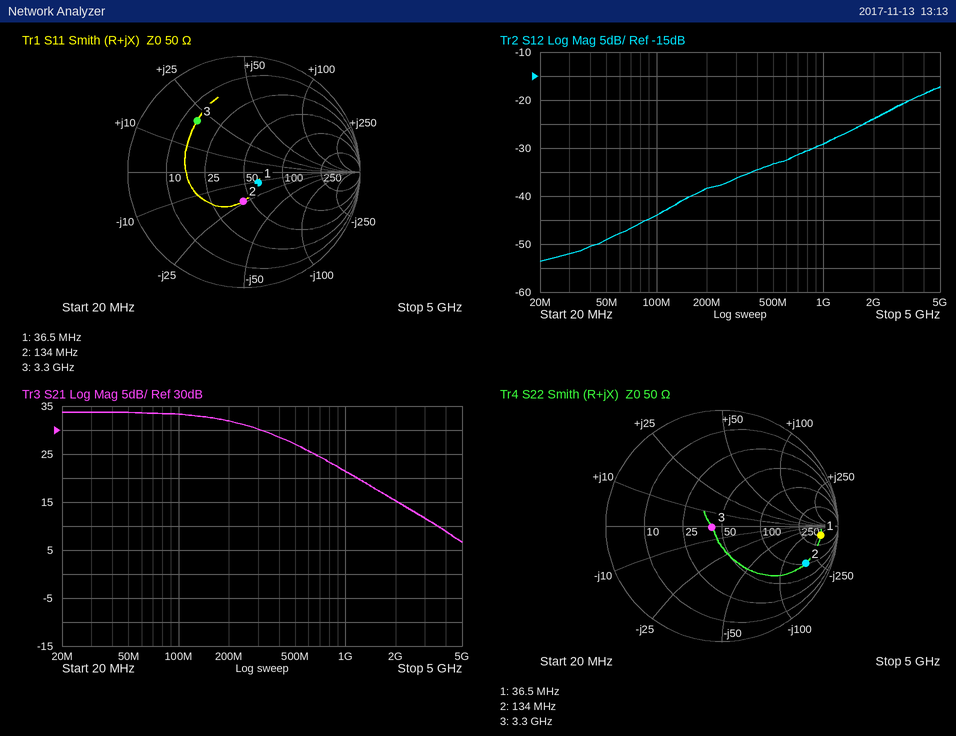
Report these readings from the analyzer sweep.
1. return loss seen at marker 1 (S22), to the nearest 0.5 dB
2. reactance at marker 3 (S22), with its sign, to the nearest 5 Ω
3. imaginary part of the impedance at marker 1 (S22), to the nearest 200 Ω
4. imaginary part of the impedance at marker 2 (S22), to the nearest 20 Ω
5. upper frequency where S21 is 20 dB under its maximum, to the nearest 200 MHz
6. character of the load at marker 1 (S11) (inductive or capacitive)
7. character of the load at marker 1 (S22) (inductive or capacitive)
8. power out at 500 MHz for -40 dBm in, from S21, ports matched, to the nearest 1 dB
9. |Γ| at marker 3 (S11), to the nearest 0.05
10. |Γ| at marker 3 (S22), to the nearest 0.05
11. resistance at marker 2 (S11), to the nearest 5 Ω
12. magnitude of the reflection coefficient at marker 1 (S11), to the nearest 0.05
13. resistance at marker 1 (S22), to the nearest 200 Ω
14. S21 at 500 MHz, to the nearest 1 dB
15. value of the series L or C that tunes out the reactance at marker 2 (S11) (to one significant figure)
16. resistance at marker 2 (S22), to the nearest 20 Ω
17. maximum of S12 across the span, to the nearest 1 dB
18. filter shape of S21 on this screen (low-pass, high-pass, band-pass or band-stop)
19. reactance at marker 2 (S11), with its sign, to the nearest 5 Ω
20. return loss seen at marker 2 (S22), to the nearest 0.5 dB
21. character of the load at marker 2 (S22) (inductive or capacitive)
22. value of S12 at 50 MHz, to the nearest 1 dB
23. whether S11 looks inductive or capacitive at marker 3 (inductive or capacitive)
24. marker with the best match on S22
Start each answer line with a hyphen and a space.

- 1.5 dB
- 0 Ω
- -200 Ω
- -180 Ω
- 2.4 GHz
- capacitive
- capacitive
- -13 dBm
- 0.60
- 0.10
- 45 Ω
- 0.15
- 400 Ω
- 27 dB
- 30 nH
- 100 Ω
- -17 dB
- low-pass
- -25 Ω
- 2.0 dB
- capacitive
- -49 dB
- inductive
- marker 3
